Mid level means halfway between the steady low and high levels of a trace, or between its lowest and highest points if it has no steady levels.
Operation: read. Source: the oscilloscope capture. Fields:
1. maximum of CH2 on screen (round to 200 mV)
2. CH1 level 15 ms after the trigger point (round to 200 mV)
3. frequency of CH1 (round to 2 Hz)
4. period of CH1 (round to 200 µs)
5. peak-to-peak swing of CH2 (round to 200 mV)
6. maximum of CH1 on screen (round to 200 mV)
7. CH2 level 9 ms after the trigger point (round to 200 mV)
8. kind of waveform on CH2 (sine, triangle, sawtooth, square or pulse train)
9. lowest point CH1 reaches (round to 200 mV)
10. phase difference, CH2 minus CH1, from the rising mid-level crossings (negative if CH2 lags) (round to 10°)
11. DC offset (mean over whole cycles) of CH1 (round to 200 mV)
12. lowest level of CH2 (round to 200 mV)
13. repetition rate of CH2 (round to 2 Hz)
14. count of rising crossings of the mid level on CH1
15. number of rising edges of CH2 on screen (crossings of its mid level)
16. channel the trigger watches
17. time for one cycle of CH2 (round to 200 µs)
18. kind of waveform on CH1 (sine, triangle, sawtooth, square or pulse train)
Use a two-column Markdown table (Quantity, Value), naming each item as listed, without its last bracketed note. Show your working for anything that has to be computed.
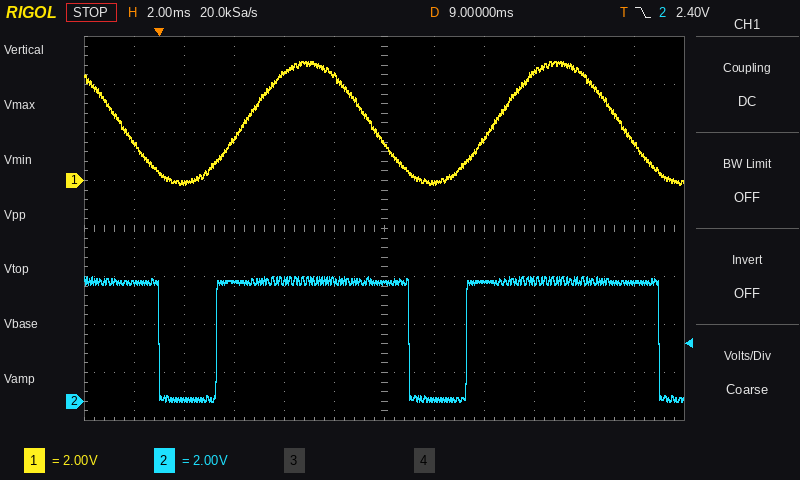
| Quantity | Value |
|---|---|
| maximum of CH2 on screen | 5.2 V |
| CH1 level 15 ms after the trigger point | 4.6 V |
| frequency of CH1 | 1 / 10.0 ms ≈ 100 Hz |
| period of CH1 | 10.0 ms |
| peak-to-peak swing of CH2 | 5.2 V − (0.0 V) = 5.2 V |
| maximum of CH1 on screen | 5.0 V |
| CH2 level 9 ms after the trigger point | 5.0 V |
| kind of waveform on CH2 | pulse train |
| lowest point CH1 reaches | -200 mV |
| phase difference, CH2 minus CH1, from the rising mid-level crossings (negative if CH2 lags) | +40° |
| DC offset (mean over whole cycles) of CH1 | (5.0 V + (-200 mV)) / 2 ≈ 2.4 V |
| lowest level of CH2 | 0.0 V |
| repetition rate of CH2 | 1 / 10.0 ms ≈ 100 Hz |
| count of rising crossings of the mid level on CH1 | 2 |
| number of rising edges of CH2 on screen | 2 |
| channel the trigger watches | CH2 |
| time for one cycle of CH2 | 10.0 ms |
| kind of waveform on CH1 | sine |
